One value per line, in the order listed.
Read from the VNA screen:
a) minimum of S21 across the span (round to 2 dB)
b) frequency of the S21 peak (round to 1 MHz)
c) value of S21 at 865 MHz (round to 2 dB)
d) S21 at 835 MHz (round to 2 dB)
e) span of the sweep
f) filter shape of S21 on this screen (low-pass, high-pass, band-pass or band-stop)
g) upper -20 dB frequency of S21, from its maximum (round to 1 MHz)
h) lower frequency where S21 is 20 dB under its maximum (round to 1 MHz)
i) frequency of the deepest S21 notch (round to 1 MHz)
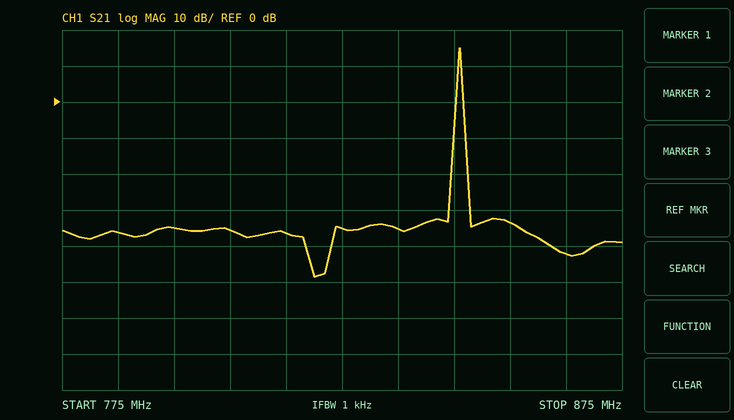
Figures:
-48 dB
846 MHz
-42 dB
-36 dB
100 MHz
band-pass
847 MHz
845 MHz
820 MHz
